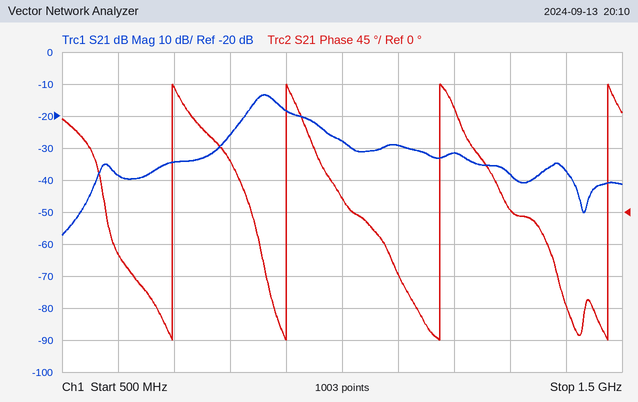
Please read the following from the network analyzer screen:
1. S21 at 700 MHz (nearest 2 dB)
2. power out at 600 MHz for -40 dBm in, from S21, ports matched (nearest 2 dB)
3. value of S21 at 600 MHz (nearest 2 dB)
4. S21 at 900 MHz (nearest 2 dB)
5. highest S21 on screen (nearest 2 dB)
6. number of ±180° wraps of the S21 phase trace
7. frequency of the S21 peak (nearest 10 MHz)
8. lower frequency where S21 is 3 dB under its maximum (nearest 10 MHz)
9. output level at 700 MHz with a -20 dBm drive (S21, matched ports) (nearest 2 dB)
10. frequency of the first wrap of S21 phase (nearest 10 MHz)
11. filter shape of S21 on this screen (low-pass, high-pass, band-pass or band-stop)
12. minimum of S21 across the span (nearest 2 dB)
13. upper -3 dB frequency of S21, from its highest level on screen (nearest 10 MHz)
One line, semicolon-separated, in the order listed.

-34 dB; -78 dBm; -38 dB; -18 dB; -14 dB; 4; 860 MHz; 840 MHz; -54 dBm; 700 MHz; band-pass; -58 dB; 890 MHz
